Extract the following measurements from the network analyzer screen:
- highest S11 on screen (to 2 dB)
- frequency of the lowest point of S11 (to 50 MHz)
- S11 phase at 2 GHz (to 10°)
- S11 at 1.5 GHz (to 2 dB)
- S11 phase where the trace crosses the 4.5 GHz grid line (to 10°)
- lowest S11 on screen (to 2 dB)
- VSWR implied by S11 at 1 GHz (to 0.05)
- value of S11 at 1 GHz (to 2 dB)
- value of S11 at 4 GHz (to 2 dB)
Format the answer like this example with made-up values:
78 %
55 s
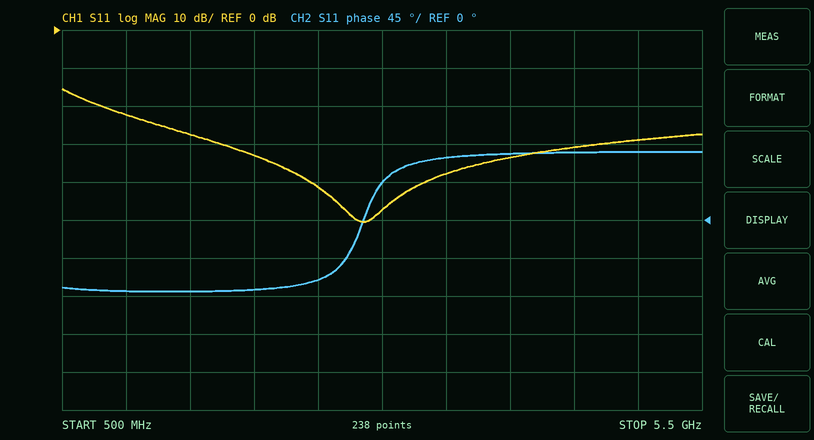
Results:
-16 dB
2.85 GHz
-80°
-28 dB
80°
-50 dB
1.15
-22 dB
-34 dB
